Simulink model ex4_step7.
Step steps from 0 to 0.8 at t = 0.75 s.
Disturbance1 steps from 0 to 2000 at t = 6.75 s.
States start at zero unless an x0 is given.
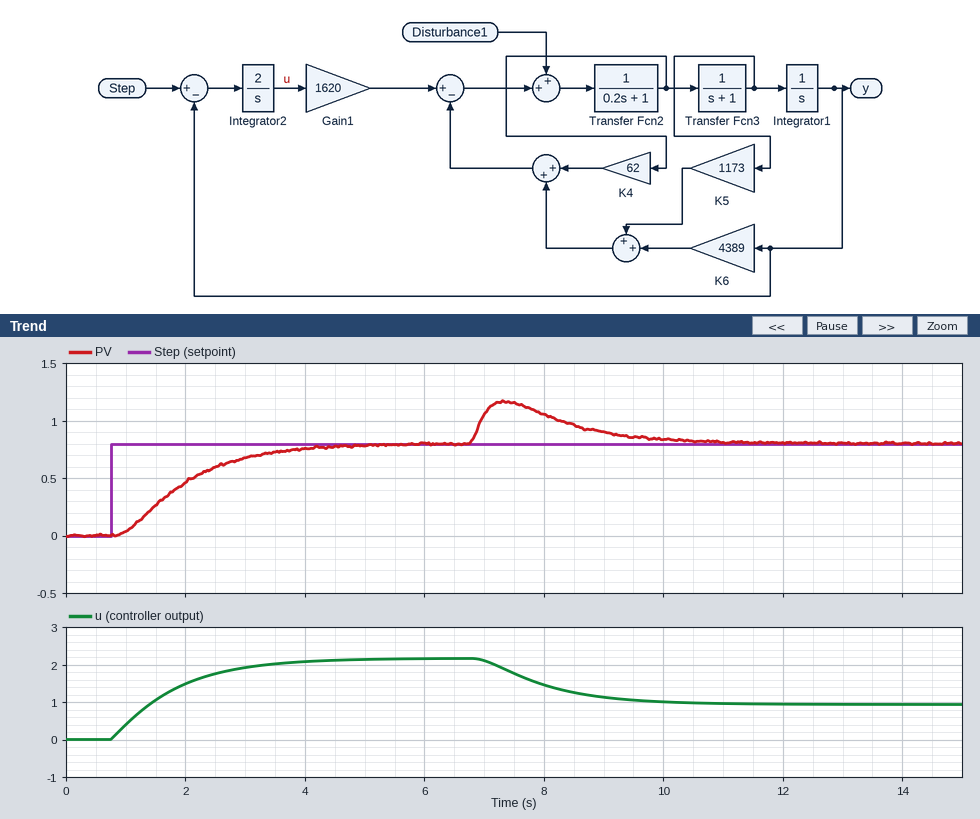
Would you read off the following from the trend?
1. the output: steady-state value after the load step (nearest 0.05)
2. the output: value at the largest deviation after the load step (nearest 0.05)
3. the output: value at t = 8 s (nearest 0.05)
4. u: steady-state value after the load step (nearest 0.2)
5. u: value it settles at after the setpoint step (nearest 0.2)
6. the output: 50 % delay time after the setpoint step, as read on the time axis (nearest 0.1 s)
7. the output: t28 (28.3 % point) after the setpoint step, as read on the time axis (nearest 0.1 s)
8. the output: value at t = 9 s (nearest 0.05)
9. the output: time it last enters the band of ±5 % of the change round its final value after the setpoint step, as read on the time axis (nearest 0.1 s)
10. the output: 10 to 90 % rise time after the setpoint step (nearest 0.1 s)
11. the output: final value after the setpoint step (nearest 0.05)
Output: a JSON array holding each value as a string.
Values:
["0.80", "1.15", "1.05", "1.0", "2.2", "1.8 s", "1.4 s", "0.90", "4.1 s", "2.3 s", "0.80"]
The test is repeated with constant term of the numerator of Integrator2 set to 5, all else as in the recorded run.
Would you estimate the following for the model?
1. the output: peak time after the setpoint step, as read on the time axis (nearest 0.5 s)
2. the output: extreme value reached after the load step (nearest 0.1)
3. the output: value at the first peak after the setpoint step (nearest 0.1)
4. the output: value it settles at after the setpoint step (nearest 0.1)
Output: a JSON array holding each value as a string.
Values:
["2.5 s", "1.1", "0.8", "0.8"]
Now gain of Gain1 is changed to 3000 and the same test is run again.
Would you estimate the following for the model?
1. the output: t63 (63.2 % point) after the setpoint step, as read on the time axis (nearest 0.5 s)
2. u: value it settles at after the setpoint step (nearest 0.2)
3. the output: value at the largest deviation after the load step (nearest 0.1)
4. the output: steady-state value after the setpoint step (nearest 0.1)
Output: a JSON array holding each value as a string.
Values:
["1.5 s", "1.2", "1.1", "0.8"]
